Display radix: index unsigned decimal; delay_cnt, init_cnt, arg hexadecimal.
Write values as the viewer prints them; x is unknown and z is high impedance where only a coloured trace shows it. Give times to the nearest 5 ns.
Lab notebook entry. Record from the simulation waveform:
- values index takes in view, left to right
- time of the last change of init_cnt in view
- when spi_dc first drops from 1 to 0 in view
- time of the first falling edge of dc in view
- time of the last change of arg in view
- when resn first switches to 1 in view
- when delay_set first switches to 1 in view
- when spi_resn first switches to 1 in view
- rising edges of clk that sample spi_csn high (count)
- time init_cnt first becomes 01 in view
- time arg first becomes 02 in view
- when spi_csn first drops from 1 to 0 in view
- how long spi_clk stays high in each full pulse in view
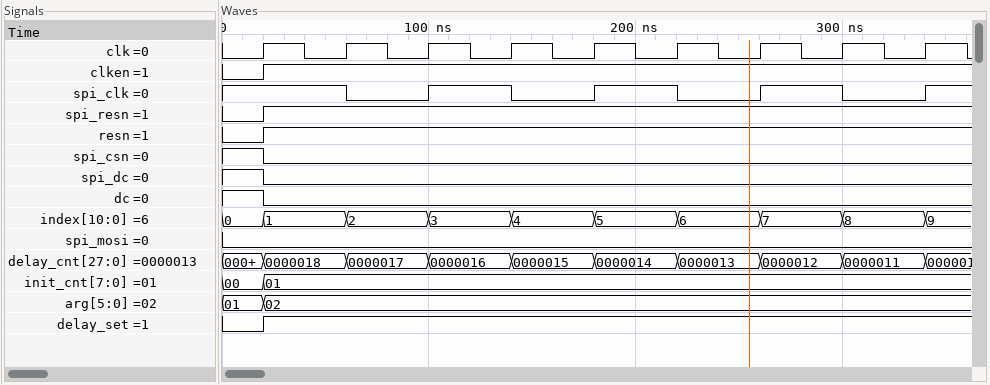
0, 1, 2, 3, 4, 5, 6, 7, 8, 9
20 ns
20 ns
20 ns
20 ns
20 ns
20 ns
20 ns
1
20 ns
20 ns
20 ns
40 ns, 40 ns, 40 ns
